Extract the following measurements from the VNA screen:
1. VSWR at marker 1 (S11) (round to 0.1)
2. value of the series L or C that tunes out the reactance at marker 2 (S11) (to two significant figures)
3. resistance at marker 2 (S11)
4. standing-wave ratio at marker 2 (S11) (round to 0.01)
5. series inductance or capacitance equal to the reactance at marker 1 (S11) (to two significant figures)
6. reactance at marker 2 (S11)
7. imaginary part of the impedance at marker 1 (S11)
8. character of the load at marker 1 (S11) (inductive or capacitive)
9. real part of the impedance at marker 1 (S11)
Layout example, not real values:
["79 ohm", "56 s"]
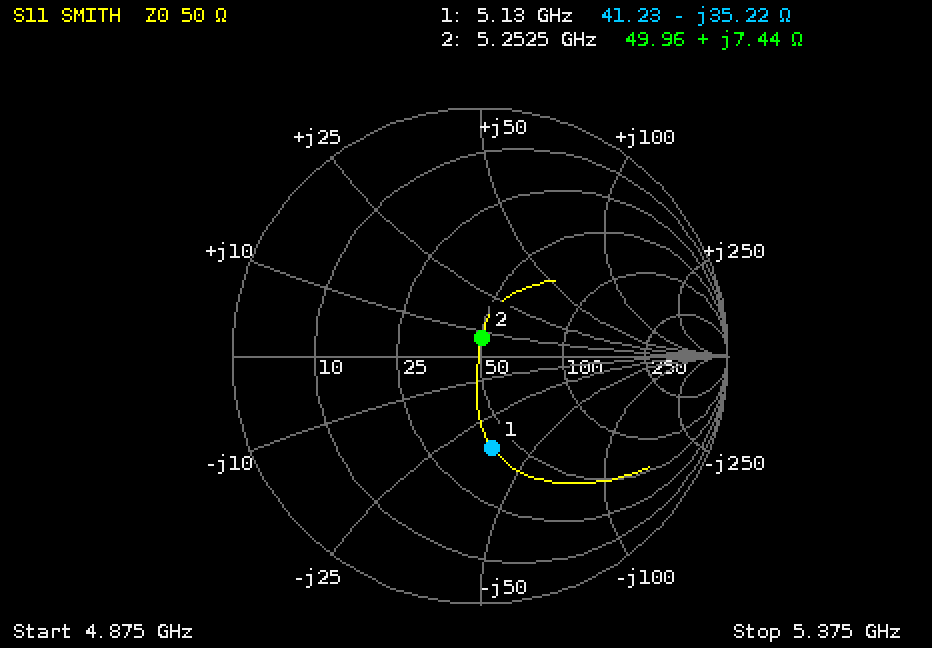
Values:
["2.2", "4.1 pF", "49.96 Ω", "1.16", "880 fF", "+7.44 Ω", "-35.22 Ω", "capacitive", "41.23 Ω"]
